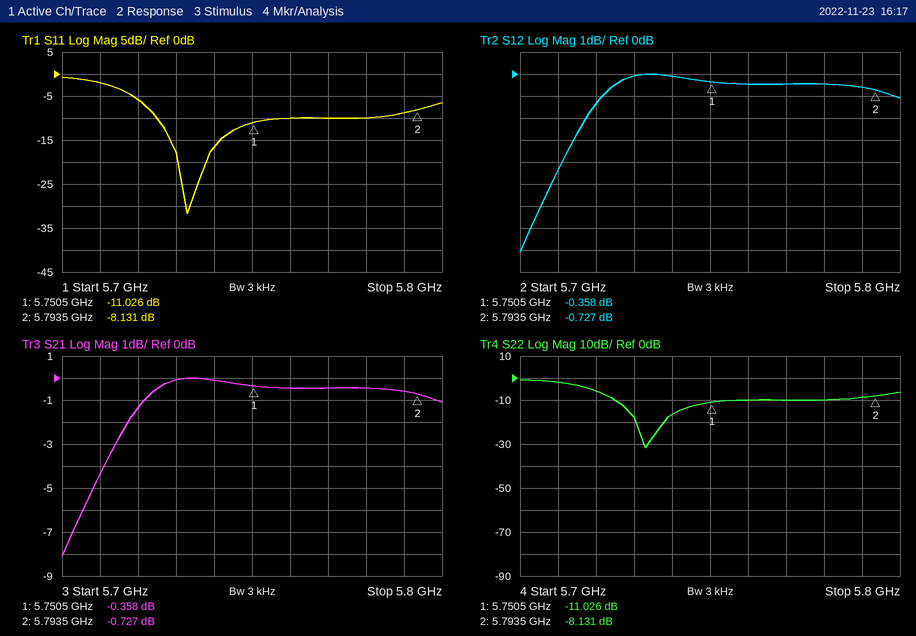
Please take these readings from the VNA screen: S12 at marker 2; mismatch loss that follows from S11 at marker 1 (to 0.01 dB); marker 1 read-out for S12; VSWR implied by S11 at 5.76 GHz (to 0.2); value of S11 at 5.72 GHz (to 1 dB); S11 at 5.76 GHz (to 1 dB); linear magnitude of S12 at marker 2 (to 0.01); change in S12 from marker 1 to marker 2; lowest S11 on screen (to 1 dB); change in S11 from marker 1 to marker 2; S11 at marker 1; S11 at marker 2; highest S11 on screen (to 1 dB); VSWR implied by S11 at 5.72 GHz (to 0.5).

-0.727 dB
0.36 dB
-0.358 dB
2.0
-6 dB
-10 dB
0.92
-0.369 dB
-32 dB
2.895 dB
-11.026 dB
-8.131 dB
-1 dB
3.0
